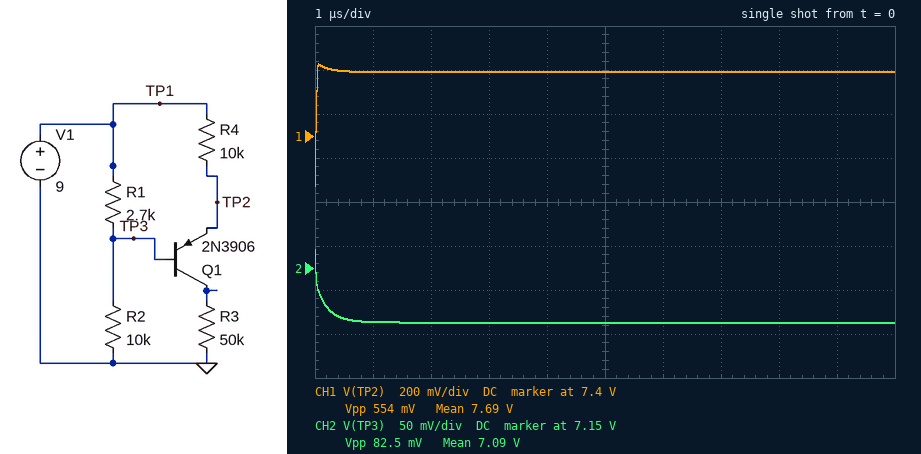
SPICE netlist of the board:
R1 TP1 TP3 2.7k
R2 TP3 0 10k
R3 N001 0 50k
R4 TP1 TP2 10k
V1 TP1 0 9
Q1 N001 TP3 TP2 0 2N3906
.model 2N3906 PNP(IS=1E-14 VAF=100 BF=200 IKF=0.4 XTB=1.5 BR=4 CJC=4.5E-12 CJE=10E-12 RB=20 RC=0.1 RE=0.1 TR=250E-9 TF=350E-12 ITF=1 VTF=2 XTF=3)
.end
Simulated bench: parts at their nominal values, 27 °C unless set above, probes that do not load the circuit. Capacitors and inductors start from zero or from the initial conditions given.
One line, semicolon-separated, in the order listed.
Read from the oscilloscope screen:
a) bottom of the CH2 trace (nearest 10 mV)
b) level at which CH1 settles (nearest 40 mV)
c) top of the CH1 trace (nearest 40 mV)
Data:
7.09 V; 7.68 V; 7.72 V
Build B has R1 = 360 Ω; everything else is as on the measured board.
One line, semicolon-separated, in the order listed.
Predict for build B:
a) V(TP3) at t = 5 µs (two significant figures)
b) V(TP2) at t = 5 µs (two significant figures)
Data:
8.7 V; 9.0 V
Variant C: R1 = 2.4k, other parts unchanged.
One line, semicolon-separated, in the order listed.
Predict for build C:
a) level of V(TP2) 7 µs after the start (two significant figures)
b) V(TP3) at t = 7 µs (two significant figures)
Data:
7.9 V; 7.3 V
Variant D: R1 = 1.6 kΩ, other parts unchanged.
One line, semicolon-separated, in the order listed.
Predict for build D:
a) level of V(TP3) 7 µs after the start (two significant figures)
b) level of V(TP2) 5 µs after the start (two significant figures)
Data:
7.8 V; 8.3 V
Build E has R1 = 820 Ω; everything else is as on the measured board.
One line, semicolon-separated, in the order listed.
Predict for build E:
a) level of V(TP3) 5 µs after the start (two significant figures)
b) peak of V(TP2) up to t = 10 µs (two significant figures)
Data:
8.3 V; 8.9 V
